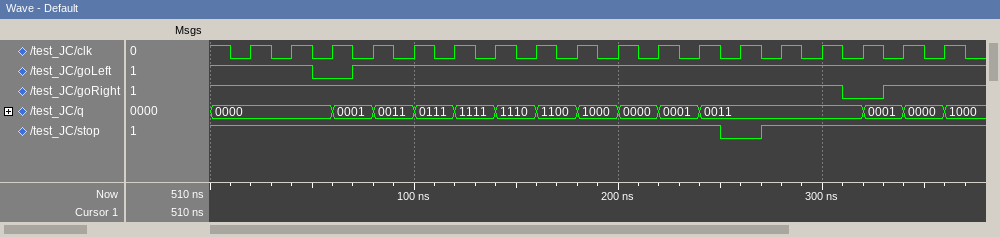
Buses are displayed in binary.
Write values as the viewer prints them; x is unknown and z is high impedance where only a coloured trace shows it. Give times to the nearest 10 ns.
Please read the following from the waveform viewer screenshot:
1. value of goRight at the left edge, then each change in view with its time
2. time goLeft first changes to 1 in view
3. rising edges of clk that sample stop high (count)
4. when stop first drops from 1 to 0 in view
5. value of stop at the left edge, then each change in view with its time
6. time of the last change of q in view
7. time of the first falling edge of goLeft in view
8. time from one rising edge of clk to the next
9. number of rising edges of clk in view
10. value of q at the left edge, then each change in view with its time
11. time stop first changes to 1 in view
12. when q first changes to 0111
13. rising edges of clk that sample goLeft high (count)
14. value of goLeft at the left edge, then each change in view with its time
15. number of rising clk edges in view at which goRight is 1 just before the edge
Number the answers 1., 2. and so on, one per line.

1. 1, 0 at 310 ns, 1 at 330 ns
2. 70 ns
3. 17
4. 250 ns
5. 1, 0 at 250 ns, 1 at 270 ns
6. 360 ns
7. 50 ns
8. 20 ns
9. 18
10. 0000, 0001 at 60 ns, 0011 at 80 ns, 0111 at 100 ns, 1111 at 120 ns, 1110 at 140 ns, 1100 at 160 ns, 1000 at 180 ns, 0000 at 200 ns, 0001 at 220 ns, 0011 at 240 ns, 0001 at 320 ns, 0000 at 340 ns, 1000 at 360 ns
11. 270 ns
12. 100 ns
13. 17
14. 1, 0 at 50 ns, 1 at 70 ns
15. 17
